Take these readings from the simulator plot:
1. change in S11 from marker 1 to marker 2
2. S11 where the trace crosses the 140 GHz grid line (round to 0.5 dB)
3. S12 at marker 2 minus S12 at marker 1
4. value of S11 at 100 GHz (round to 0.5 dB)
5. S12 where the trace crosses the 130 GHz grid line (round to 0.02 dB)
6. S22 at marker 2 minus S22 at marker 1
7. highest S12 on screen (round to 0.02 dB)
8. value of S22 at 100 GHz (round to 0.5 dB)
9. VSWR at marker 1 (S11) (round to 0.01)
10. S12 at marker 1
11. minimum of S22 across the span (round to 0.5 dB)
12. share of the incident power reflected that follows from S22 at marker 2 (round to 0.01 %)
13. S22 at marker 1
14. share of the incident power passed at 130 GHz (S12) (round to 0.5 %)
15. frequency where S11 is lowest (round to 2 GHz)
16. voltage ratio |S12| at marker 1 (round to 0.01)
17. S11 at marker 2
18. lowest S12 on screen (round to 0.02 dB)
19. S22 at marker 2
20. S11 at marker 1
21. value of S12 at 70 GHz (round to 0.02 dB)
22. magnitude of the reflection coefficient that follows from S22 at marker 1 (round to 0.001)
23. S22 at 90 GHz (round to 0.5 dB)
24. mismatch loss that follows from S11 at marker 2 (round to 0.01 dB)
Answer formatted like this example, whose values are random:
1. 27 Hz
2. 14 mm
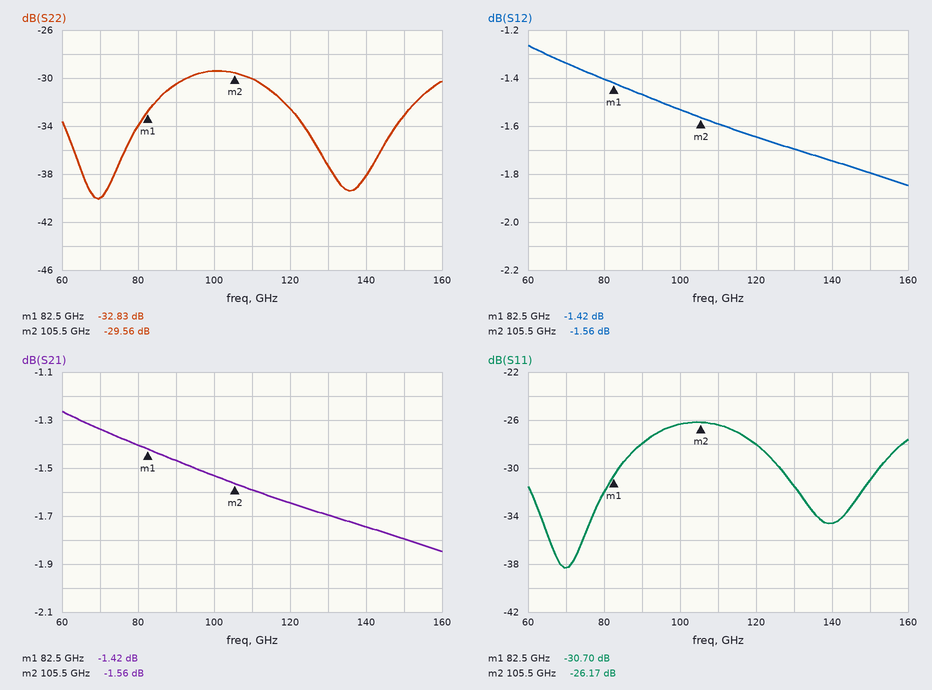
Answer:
1. 4.53 dB
2. -34.5 dB
3. -0.14 dB
4. -26.5 dB
5. -1.70 dB
6. 3.27 dB
7. -1.26 dB
8. -29.5 dB
9. 1.06
10. -1.42 dB
11. -40.0 dB
12. 0.11 %
13. -32.83 dB
14. 67.5 %
15. 70 GHz
16. 0.85
17. -26.17 dB
18. -1.84 dB
19. -29.56 dB
20. -30.70 dB
21. -1.34 dB
22. 0.023
23. -30.5 dB
24. 0.01 dB
